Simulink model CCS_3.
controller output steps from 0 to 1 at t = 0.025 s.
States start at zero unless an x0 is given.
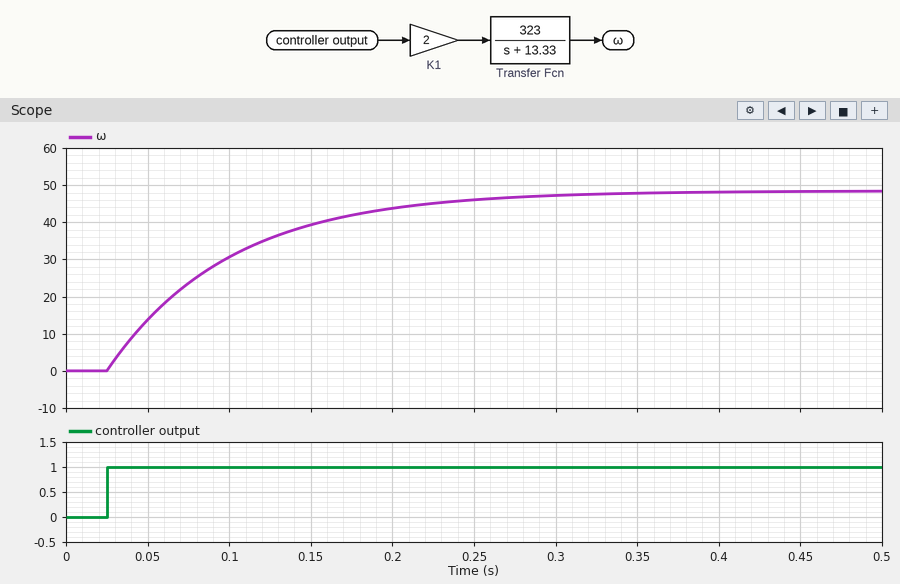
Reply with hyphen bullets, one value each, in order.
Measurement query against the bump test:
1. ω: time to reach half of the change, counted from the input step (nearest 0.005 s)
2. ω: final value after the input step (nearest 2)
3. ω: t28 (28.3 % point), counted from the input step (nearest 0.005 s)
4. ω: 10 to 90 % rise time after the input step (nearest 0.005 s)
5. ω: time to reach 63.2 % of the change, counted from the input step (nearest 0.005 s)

- 0.050 s
- 48
- 0.025 s
- 0.165 s
- 0.075 s
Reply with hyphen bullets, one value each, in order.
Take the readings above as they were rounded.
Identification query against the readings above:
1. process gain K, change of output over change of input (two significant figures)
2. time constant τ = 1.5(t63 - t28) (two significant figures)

- 48
- 0.075 s
